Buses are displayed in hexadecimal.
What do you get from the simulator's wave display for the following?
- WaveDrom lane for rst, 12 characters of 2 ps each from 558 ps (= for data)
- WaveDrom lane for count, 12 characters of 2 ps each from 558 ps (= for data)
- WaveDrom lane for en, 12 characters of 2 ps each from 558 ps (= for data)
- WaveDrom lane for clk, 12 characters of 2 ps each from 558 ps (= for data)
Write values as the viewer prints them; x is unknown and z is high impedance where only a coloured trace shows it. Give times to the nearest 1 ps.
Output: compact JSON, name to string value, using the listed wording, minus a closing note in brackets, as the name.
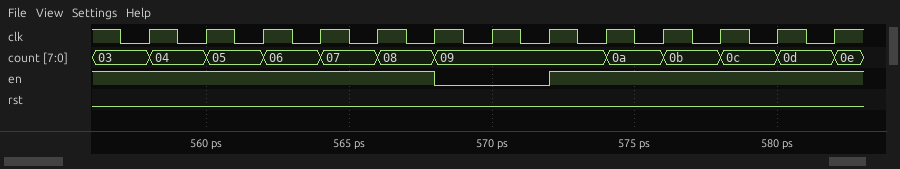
{"WaveDrom lane for rst, 12 characters of 2 ps each from 558 ps": "{name: 'rst', wave: '0...........'}", "WaveDrom lane for count, 12 characters of 2 ps each from 558 ps": "{name: 'count', wave: '======..====', data: '04 05 06 07 08 09 0a 0b 0c 0d'}", "WaveDrom lane for en, 12 characters of 2 ps each from 558 ps": "{name: 'en', wave: '1....0.1....'}", "WaveDrom lane for clk, 12 characters of 2 ps each from 558 ps": "{name: 'clk', wave: 'p...........'}"}
